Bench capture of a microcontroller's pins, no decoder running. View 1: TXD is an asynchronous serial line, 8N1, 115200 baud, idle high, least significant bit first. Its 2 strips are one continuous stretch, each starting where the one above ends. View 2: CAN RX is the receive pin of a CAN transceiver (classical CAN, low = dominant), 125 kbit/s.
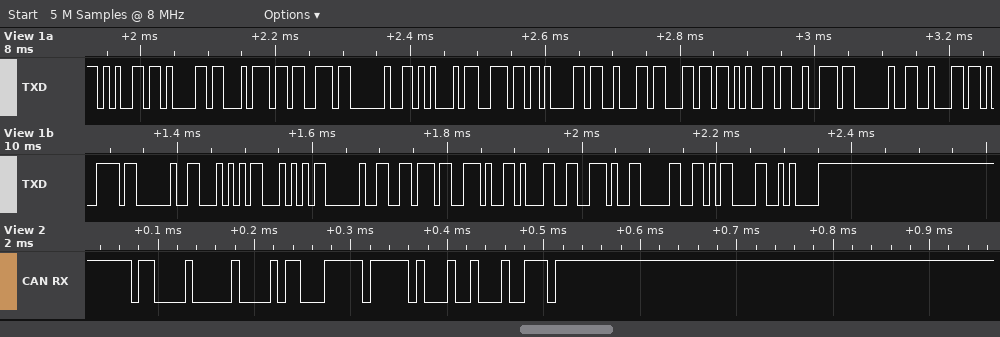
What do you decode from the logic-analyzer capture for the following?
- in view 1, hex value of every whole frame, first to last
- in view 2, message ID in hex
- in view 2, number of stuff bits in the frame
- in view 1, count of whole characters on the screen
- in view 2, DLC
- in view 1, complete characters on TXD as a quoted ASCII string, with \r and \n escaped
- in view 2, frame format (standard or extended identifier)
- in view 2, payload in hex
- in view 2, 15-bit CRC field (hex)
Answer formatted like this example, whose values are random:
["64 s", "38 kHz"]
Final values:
["65 61 74 73 20 45 6E 61 62 6C 65 72 20 62 79 20 54 54 20 76 2E 31 2E 30 0D 0A", "0x610", "3", "26", "2", "\"eats Enabler by TT v.1.0\\r\\n\"", "standard", "C7 FF", "0x0913"]
